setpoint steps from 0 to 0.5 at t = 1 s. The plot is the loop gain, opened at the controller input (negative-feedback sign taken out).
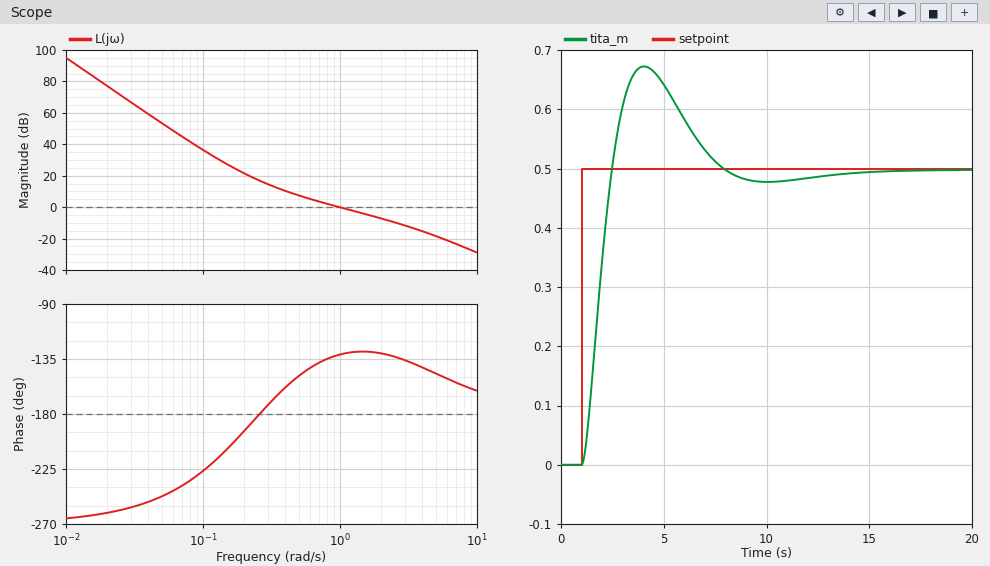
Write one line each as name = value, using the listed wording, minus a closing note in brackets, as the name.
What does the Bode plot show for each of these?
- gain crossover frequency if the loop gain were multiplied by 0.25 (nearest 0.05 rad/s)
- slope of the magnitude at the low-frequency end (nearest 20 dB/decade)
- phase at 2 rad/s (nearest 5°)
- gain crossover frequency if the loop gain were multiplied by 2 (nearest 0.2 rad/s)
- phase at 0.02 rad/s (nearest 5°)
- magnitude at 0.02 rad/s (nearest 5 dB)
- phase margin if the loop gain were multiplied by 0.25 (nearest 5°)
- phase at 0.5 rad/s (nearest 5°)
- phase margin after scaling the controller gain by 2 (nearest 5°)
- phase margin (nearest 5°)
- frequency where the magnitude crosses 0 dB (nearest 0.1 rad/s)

gain crossover frequency if the loop gain were multiplied by 0.25 = 0.35 rad/s
slope of the magnitude at the low-frequency end = -60 dB/decade
phase at 2 rad/s = -130°
gain crossover frequency if the loop gain were multiplied by 2 = 1.8 rad/s
phase at 0.02 rad/s = -260°
magnitude at 0.02 rad/s = 75 dB
phase margin if the loop gain were multiplied by 0.25 = 15°
phase at 0.5 rad/s = -150°
phase margin after scaling the controller gain by 2 = 50°
phase margin = 50°
frequency where the magnitude crosses 0 dB = 1.0 rad/s
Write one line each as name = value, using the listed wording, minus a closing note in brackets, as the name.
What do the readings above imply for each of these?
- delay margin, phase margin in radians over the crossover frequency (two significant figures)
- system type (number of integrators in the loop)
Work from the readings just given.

delay margin, phase margin in radians over the crossover frequency = 0.87 s
system type = 3
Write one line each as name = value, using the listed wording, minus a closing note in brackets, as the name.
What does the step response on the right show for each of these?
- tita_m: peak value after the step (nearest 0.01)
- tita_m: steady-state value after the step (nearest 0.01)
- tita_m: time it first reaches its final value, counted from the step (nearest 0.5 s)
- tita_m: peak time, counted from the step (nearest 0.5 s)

tita_m: peak value after the step = 0.67
tita_m: steady-state value after the step = 0.50
tita_m: time it first reaches its final value, counted from the step = 1.5 s
tita_m: peak time, counted from the step = 3.0 s
